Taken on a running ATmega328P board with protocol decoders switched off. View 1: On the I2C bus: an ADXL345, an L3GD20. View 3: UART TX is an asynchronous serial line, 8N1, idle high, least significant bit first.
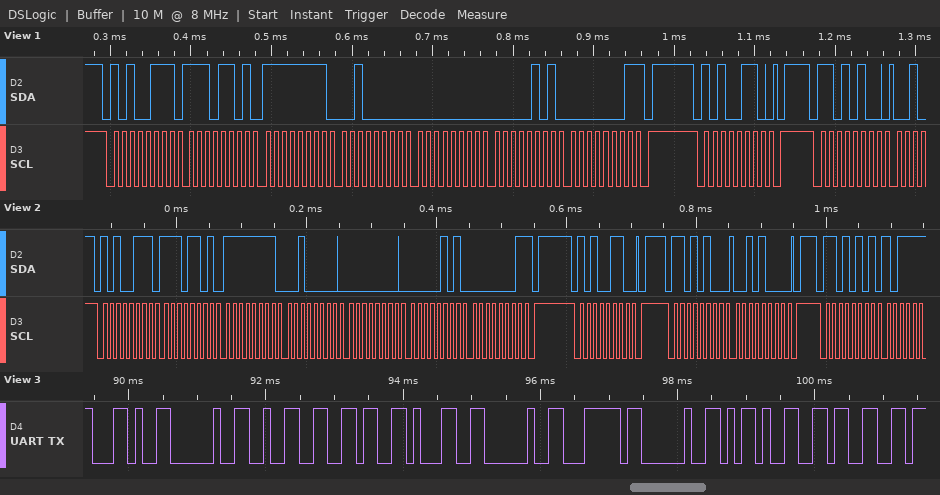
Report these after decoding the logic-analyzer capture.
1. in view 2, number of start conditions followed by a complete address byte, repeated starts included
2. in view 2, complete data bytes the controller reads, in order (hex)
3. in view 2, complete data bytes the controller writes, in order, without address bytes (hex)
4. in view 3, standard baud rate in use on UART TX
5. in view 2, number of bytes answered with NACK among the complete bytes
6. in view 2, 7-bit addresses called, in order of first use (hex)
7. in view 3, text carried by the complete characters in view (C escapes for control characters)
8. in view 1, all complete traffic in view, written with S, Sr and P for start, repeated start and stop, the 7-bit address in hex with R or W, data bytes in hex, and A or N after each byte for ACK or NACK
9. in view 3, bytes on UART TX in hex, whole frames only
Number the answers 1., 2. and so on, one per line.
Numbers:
1. 4
2. ED FF 20 00 05 01
3. 28
4. 9600 baud
5. 1
6. 0x53 0x6A
7. ", 261 | -6"
8. S 53R A ED A FF A 20 A 00 A 05 A 01 N P S 53W A P S 6AW A
9. 2C 20 32 36 31 20 7C 20 2D 36
